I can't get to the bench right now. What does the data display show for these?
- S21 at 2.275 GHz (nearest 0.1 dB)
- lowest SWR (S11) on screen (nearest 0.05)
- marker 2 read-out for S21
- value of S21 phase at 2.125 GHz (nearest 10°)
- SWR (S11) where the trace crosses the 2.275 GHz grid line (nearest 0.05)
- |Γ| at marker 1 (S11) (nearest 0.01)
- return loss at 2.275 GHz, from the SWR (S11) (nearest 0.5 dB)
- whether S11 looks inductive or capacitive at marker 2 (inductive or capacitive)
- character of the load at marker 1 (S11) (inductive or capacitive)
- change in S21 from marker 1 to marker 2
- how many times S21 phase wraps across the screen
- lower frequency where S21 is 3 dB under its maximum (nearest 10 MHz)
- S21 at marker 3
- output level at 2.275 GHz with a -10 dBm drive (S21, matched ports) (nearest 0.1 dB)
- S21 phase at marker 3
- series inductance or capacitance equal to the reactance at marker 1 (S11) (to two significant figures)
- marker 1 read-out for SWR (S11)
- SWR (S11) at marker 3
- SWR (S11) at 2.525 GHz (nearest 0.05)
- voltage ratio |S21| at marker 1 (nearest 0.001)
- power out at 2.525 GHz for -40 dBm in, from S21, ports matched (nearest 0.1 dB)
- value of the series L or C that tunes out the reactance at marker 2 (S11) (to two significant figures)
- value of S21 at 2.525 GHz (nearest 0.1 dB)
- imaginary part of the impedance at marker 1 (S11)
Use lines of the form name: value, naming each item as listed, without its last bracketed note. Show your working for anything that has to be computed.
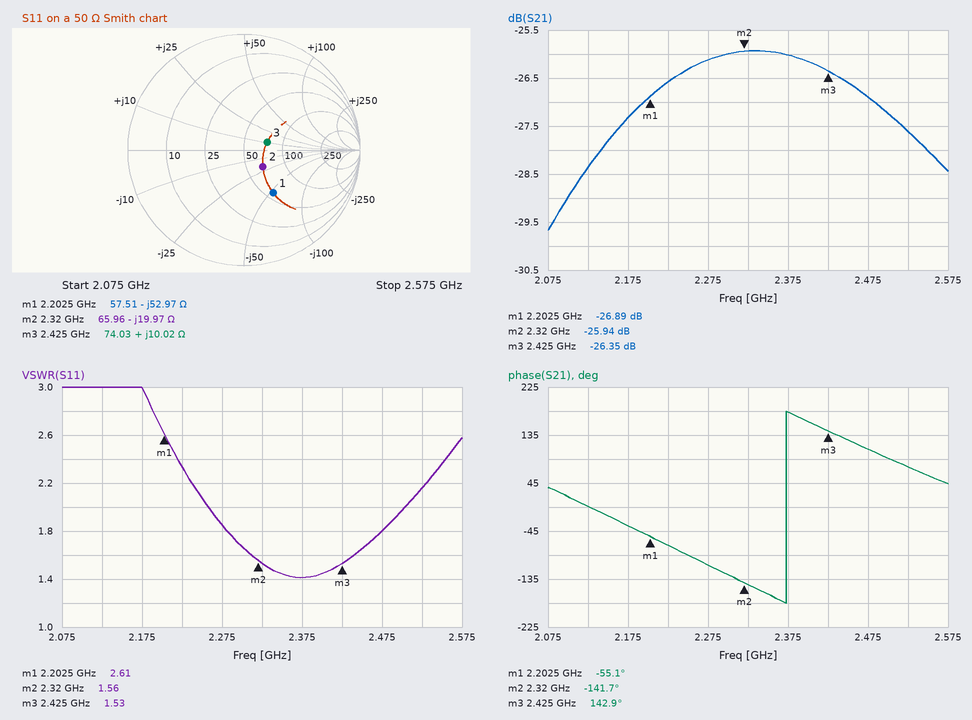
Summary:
S21 at 2.275 GHz: -26.1 dB
lowest SWR (S11) on screen: 1.40
marker 2 read-out for S21: -25.94 dB
value of S21 phase at 2.125 GHz: 0°
SWR (S11) where the trace crosses the 2.275 GHz grid line: 1.85
|Γ| at marker 1 (S11): 0.45
return loss at 2.275 GHz, from the SWR (S11): −20 log10((1.85 − 1)/(1.85 + 1)) ≈ 10.5 dB
whether S11 looks inductive or capacitive at marker 2: capacitive
character of the load at marker 1 (S11): capacitive
change in S21 from marker 1 to marker 2: -25.94 − (-26.89) = 0.95 dB
how many times S21 phase wraps across the screen: 1
lower frequency where S21 is 3 dB under its maximum: 2.10 GHz
S21 at marker 3: -26.35 dB
output level at 2.275 GHz with a -10 dBm drive (S21, matched ports): -10 dBm + (-26.1 dB) = -36.1 dBm
S21 phase at marker 3: 142.9°
series inductance or capacitance equal to the reactance at marker 1 (S11): C = 1/(2π × 2.2025 GHz × 52.97 Ω) ≈ 1.4 pF
marker 1 read-out for SWR: 2.61
SWR (S11) at marker 3: 1.53
SWR (S11) at 2.525 GHz: 2.15
voltage ratio |S21| at marker 1: 10^(-26.89/20) ≈ 0.045
power out at 2.525 GHz for -40 dBm in, from S21, ports matched: -40 dBm + (-27.6 dB) = -67.6 dBm
value of the series L or C that tunes out the reactance at marker 2 (S11): L = 19.97 Ω/(2π × 2.32 GHz) ≈ 1.4 nH
value of S21 at 2.525 GHz: -27.6 dB
imaginary part of the impedance at marker 1: -52.97 Ω
